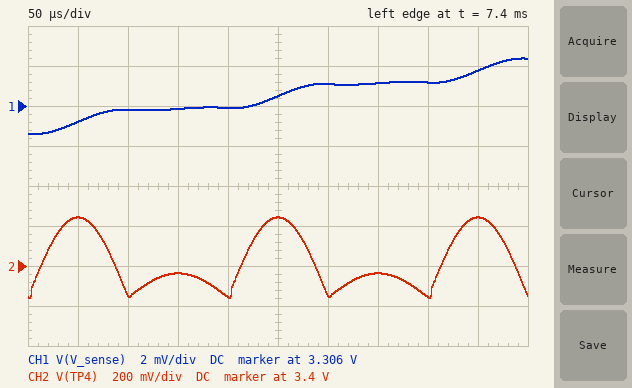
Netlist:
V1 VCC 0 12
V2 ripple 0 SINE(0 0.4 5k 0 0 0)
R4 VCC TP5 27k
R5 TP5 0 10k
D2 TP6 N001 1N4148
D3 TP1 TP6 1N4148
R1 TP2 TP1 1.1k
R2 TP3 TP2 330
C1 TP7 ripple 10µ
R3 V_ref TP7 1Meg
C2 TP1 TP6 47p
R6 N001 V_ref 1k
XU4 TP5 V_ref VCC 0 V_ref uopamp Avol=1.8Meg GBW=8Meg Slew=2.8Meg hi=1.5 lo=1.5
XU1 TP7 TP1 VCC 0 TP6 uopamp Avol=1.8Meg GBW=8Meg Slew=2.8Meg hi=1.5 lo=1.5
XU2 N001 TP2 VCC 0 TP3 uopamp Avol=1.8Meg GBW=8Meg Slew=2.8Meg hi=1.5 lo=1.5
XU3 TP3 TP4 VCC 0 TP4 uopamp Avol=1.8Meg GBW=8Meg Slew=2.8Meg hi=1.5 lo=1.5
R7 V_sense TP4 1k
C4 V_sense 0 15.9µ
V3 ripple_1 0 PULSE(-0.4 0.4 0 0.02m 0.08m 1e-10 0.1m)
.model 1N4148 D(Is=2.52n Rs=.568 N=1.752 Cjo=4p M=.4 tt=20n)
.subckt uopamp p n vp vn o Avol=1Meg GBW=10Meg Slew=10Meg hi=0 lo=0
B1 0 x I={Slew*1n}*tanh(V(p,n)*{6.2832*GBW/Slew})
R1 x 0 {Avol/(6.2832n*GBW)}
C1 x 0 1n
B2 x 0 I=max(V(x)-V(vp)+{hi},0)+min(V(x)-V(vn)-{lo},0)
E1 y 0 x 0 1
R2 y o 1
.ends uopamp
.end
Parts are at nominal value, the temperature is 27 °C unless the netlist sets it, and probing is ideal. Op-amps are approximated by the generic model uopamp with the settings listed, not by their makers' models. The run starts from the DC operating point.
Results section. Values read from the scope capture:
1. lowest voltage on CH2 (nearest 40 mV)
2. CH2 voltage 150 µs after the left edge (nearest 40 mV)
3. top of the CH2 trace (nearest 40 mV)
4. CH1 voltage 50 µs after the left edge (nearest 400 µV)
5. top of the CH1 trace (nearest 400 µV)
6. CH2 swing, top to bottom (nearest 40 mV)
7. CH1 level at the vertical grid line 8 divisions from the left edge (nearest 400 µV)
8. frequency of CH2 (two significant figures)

3.24 V
3.36 V
3.64 V
3.3052 V
3.3084 V
400 mV
3.3072 V
5.0 kHz
